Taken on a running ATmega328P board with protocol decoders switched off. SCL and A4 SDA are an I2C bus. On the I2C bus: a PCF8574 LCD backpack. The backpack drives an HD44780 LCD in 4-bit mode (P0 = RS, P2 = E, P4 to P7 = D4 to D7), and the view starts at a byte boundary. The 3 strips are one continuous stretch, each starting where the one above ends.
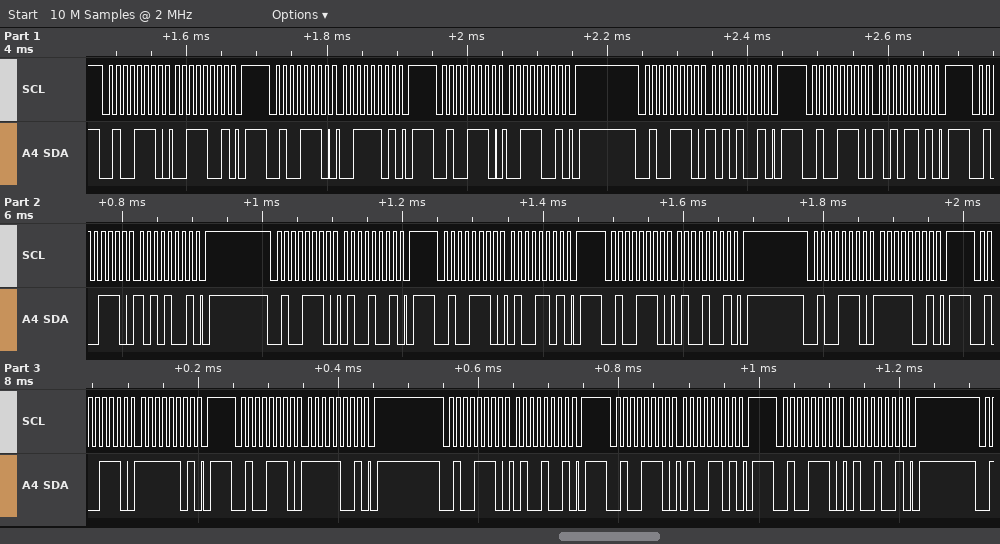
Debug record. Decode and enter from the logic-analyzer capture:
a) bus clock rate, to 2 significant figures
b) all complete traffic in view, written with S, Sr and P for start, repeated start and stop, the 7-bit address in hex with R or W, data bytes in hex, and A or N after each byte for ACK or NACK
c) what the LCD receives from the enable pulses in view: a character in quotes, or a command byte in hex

100 kHz
S 27W A 39 A P S 27W A 3D A P S 27W A 39 A P S 27W A A9 A P S 27W A AD A P S 27W A A9 A P S 27W A 49 A P S 27W A 4D A P S 27W A 49 A P S 27W A F9 A P S 27W A FD A P S 27W A F9 A P S 27W A 49 A P S 27W A 4D A P S 27W A 49 A P
':' 'O'
